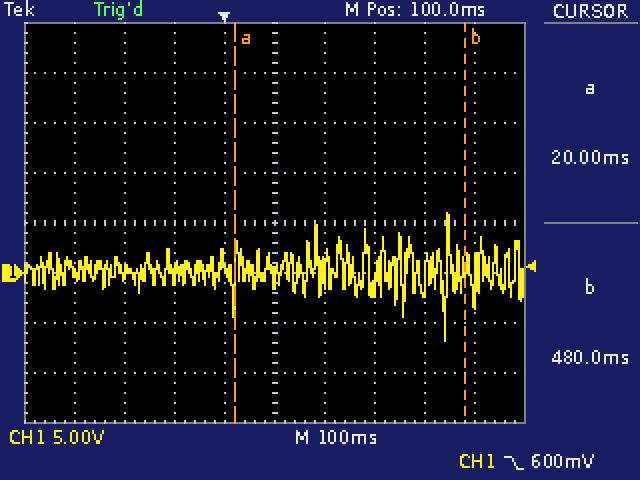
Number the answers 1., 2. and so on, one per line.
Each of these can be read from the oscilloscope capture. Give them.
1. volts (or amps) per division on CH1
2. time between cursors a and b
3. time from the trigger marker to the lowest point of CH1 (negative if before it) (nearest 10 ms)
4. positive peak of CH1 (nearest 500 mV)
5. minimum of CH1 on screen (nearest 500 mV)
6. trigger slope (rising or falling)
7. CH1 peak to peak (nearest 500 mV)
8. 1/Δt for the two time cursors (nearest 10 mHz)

1. 5 V
2. 460 ms
3. +440 ms
4. 6.0 V
5. -7.0 V
6. falling
7. 13.0 V
8. 2.17 Hz
